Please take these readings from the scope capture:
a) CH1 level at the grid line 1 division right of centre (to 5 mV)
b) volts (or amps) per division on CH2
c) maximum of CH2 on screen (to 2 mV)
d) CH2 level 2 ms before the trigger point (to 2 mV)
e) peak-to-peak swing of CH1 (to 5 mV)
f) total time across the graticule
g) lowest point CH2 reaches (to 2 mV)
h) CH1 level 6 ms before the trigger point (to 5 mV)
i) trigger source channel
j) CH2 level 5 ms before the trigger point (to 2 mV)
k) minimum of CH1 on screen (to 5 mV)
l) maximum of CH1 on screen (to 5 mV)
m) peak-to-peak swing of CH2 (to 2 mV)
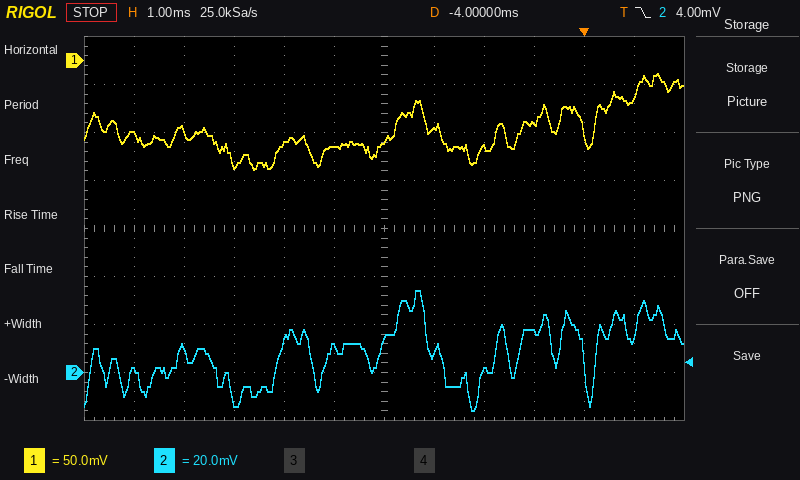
-70 mV
20 mV
34 mV
0 mV
100 mV
12 ms
-16 mV
-85 mV
CH2
10 mV
-115 mV
-15 mV
50 mV
